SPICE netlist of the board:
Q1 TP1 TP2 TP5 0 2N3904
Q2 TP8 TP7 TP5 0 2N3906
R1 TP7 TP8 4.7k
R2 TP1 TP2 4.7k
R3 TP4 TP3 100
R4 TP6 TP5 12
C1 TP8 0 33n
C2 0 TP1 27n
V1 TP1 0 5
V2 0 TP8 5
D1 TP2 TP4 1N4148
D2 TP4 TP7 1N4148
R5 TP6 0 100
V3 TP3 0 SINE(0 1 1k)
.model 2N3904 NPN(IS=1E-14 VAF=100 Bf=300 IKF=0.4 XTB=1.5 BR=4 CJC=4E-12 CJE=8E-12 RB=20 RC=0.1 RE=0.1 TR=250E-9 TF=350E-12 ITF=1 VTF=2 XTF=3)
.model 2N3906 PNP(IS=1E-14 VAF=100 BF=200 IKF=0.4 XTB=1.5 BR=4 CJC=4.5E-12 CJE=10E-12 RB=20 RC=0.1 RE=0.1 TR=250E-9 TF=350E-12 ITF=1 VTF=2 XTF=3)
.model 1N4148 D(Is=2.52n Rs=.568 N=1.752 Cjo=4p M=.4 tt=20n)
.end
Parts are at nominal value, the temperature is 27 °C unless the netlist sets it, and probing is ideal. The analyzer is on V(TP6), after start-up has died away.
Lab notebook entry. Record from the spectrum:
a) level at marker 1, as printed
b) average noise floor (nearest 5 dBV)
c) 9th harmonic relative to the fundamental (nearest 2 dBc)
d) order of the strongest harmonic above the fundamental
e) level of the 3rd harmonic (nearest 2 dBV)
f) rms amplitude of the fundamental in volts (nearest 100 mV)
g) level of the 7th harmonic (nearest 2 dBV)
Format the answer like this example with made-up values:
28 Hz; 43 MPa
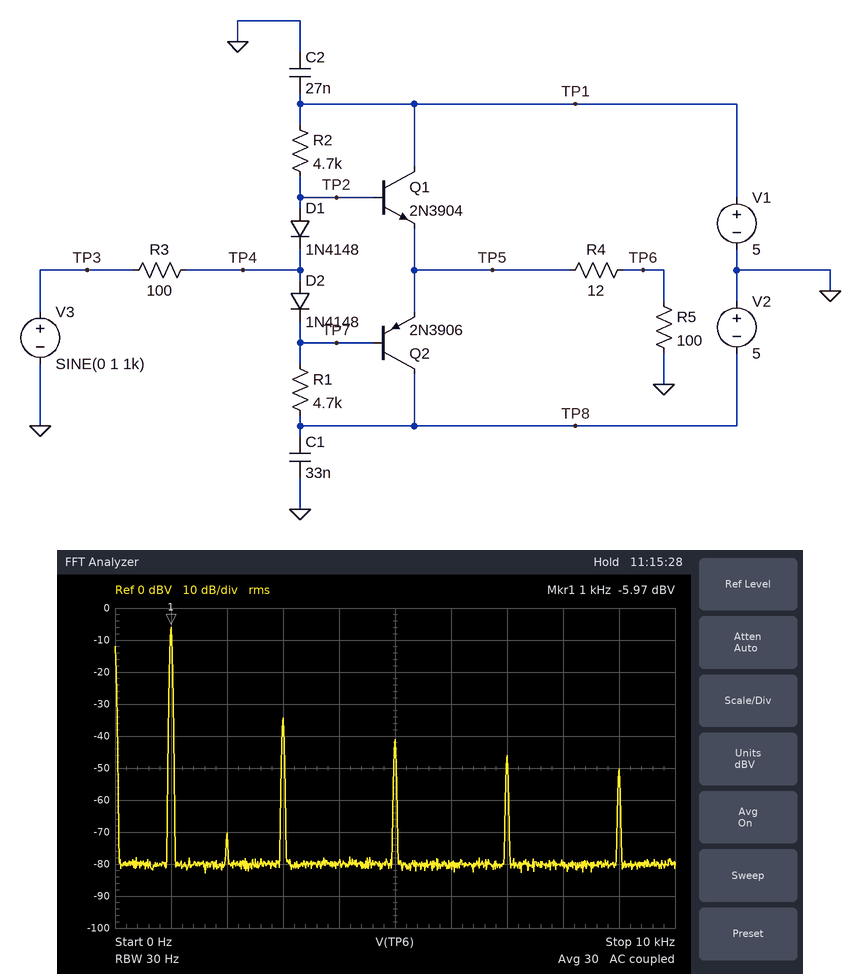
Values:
-5.97 dBV; -80 dBV; -44 dBc; 3; -34 dBV; 500 mV; -46 dBV
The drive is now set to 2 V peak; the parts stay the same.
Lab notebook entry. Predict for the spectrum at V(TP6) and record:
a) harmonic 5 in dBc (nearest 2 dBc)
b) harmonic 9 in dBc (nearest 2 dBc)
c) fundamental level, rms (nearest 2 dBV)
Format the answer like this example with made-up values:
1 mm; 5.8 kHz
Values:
-38 dBc; -46 dBc; 0 dBV
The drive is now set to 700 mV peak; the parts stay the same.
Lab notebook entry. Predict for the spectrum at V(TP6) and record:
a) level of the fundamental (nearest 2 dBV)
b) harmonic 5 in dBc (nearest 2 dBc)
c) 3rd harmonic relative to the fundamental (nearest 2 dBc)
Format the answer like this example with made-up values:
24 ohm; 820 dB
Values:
-10 dBV; -34 dBc; -26 dBc
